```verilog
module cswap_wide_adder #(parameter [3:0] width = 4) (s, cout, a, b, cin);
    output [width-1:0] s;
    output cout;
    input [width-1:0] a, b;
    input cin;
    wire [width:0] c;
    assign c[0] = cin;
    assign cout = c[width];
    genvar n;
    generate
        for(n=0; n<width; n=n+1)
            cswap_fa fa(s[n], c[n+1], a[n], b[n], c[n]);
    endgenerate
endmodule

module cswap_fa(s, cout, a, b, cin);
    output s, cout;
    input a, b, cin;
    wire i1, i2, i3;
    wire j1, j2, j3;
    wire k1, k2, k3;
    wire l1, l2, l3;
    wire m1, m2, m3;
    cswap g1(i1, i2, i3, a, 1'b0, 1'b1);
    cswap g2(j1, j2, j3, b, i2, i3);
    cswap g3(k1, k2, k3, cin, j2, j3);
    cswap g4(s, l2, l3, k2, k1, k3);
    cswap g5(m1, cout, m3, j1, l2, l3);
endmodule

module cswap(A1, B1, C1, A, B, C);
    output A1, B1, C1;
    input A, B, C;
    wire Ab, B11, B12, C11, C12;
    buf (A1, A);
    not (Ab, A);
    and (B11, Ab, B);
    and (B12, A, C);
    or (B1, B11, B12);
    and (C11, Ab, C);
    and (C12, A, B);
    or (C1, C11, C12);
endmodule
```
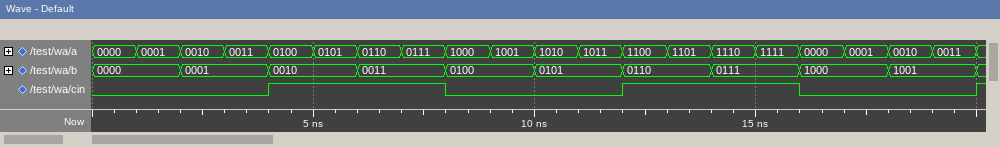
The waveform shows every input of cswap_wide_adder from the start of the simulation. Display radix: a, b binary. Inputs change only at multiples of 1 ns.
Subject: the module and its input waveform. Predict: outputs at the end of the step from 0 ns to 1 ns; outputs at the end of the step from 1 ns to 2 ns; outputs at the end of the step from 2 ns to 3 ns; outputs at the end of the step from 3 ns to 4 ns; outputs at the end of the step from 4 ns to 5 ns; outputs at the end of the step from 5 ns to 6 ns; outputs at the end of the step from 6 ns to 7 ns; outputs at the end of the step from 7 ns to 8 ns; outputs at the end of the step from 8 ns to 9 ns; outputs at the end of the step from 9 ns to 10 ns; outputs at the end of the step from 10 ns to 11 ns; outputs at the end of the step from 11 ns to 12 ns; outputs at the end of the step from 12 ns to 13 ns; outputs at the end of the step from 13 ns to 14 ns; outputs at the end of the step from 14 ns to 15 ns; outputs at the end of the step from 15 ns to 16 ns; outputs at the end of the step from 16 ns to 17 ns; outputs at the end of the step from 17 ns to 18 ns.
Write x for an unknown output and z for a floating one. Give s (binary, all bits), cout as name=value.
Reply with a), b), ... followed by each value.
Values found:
a) s=0000, cout=0
b) s=0001, cout=0
c) s=0011, cout=0
d) s=0100, cout=0
e) s=0111, cout=0
f) s=1000, cout=0
g) s=1010, cout=0
h) s=1011, cout=0
i) s=1100, cout=0
j) s=1101, cout=0
k) s=1111, cout=0
l) s=0000, cout=1
m) s=0011, cout=1
n) s=0100, cout=1
o) s=0110, cout=1
p) s=0111, cout=1
q) s=1000, cout=0
r) s=1001, cout=0
